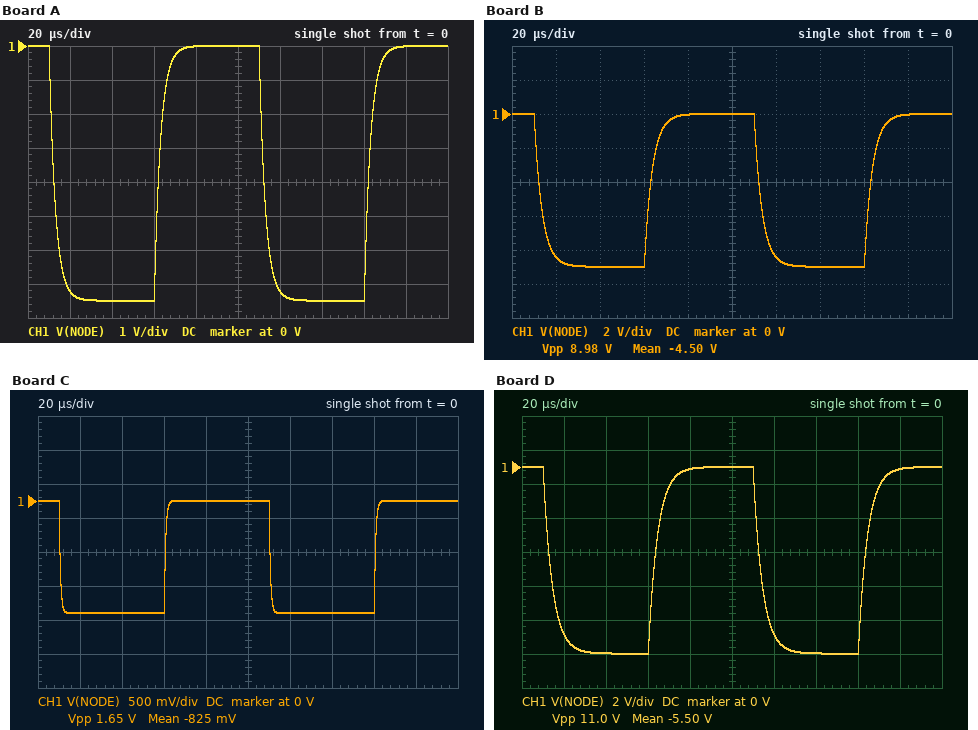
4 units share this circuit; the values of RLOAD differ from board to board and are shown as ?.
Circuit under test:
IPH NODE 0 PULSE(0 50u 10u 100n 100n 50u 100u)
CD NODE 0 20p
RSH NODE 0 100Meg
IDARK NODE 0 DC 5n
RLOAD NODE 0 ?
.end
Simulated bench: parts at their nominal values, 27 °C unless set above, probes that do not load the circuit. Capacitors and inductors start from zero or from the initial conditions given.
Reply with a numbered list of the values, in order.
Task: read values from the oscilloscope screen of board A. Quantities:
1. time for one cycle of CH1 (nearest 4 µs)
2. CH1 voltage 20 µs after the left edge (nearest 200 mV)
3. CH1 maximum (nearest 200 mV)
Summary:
1. 100 µs
2. -7.2 V
3. 0 V
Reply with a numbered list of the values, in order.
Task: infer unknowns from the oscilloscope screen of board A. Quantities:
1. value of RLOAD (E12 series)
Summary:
1. 150 kΩ
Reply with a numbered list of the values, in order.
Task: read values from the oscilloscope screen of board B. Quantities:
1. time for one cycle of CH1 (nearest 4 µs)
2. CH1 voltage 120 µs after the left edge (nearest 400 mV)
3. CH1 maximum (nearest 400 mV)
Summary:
1. 100 µs
2. -8.4 V
3. 0 V
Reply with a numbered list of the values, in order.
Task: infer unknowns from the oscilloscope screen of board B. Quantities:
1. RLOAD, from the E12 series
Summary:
1. 180 kΩ
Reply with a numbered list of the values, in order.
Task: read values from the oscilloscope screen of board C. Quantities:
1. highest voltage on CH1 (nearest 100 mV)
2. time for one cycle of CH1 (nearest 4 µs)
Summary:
1. 0 V
2. 100 µs
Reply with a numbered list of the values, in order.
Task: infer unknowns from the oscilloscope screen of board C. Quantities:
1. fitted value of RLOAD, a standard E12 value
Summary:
1. 33 kΩ
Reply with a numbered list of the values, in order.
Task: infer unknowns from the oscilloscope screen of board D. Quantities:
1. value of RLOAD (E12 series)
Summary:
1. 220 kΩ
